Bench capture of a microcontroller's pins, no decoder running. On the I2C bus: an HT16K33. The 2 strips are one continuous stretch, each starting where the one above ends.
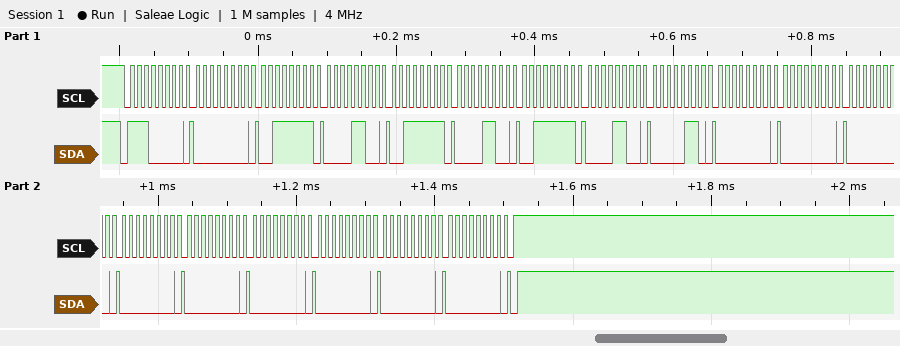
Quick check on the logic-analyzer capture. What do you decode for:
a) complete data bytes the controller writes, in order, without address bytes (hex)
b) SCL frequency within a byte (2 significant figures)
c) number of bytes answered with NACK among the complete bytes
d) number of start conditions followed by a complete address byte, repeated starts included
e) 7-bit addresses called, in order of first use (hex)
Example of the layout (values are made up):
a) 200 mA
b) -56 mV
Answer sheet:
a) 00 3F 0C 3F 0C 3F 0C 06 00 00 00 00 00 00 00 00 00
b) 100 kHz
c) 0
d) 1
e) 0x70
